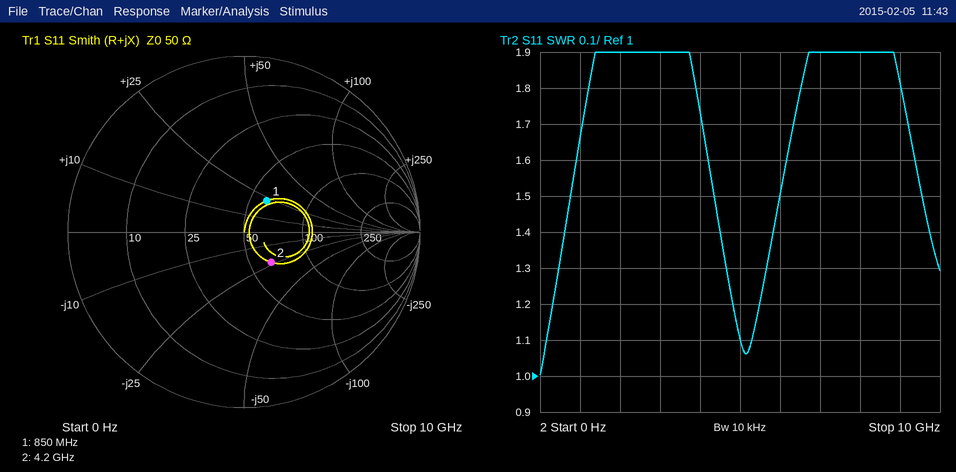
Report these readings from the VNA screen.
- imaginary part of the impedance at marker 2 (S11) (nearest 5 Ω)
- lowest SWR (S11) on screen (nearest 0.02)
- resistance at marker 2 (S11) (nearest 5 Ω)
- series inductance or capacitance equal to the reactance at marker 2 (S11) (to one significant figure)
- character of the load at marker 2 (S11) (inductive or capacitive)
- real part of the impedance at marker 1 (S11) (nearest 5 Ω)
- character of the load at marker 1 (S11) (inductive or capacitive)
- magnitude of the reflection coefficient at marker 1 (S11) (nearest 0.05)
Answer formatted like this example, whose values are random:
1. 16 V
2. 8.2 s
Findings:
1. -25 Ω
2. 1.00
3. 65 Ω
4. 2 pF
5. capacitive
6. 60 Ω
7. inductive
8. 0.20
